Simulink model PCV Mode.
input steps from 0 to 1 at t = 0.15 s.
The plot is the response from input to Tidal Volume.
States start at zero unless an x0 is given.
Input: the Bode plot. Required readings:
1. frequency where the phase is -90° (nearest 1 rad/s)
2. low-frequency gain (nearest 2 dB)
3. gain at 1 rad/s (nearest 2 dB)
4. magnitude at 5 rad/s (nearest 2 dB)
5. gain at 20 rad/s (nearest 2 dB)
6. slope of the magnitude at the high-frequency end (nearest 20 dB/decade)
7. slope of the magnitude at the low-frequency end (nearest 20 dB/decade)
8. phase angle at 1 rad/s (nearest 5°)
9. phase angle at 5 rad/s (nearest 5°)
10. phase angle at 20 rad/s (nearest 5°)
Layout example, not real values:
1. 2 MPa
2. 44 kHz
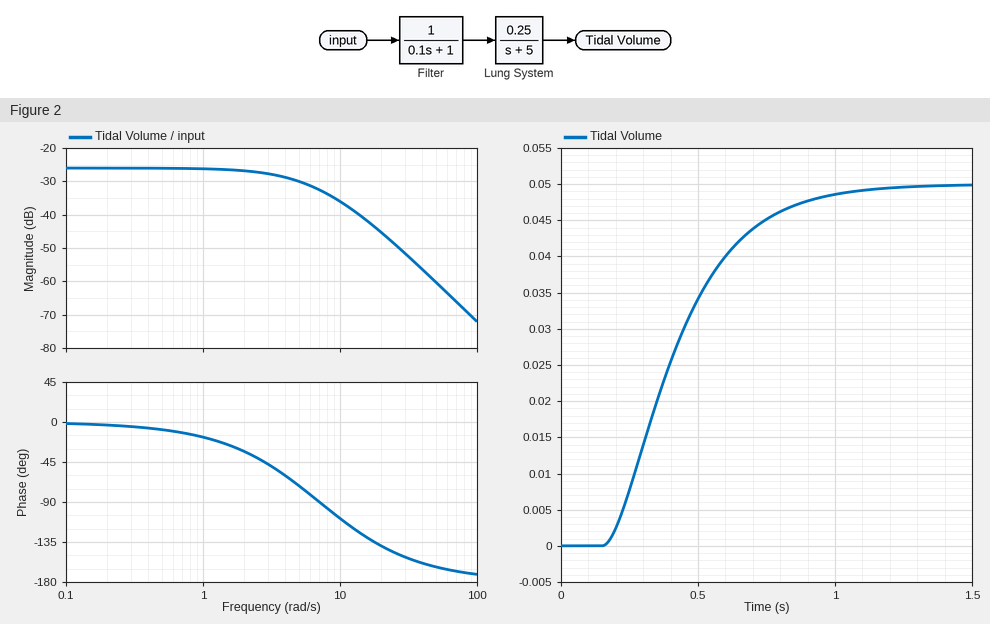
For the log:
1. 7 rad/s
2. -26 dB
3. -26 dB
4. -30 dB
5. -46 dB
6. -40 dB/decade
7. 0 dB/decade
8. -15°
9. -70°
10. -140°
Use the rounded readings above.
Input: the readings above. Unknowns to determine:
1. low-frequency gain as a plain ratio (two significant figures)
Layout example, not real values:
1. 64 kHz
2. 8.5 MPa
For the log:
1. 0.050
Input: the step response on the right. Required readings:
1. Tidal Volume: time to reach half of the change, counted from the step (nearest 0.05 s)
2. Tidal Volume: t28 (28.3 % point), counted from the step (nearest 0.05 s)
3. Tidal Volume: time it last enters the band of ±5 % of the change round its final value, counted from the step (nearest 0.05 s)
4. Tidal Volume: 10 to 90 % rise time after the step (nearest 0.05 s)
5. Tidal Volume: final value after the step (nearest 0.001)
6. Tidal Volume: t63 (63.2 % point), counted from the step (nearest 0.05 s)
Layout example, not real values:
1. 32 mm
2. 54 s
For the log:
1. 0.25 s
2. 0.15 s
3. 0.75 s
4. 0.50 s
5. 0.050
6. 0.30 s
